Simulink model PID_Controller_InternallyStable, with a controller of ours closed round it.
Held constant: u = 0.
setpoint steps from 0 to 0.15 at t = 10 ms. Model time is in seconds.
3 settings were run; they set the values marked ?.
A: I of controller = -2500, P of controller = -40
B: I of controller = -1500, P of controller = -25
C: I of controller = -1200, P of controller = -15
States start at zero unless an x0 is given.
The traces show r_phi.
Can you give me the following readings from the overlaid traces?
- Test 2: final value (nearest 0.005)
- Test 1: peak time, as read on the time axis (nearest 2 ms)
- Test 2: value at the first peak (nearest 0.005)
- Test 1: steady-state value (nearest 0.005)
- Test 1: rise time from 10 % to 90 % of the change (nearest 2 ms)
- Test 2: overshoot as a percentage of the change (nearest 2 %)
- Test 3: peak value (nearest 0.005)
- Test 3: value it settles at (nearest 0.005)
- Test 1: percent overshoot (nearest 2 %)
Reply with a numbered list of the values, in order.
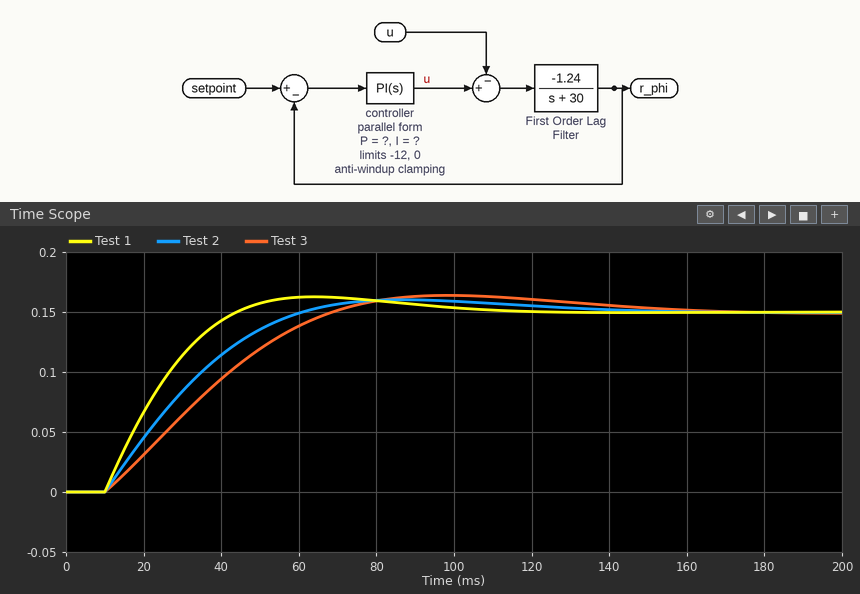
1. 0.150
2. 64 ms
3. 0.160
4. 0.150
5. 24 ms
6. 6 %
7. 0.165
8. 0.150
9. 8 %
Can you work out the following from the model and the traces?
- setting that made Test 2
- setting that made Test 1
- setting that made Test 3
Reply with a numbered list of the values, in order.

1. B
2. A
3. C
